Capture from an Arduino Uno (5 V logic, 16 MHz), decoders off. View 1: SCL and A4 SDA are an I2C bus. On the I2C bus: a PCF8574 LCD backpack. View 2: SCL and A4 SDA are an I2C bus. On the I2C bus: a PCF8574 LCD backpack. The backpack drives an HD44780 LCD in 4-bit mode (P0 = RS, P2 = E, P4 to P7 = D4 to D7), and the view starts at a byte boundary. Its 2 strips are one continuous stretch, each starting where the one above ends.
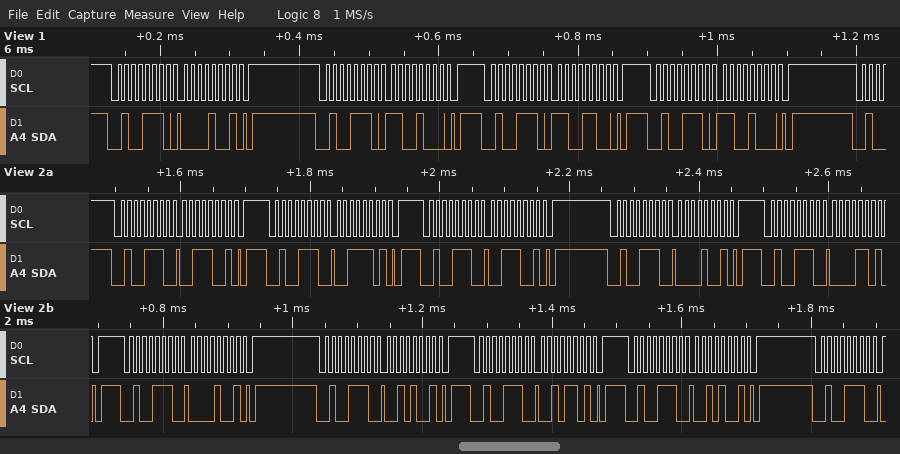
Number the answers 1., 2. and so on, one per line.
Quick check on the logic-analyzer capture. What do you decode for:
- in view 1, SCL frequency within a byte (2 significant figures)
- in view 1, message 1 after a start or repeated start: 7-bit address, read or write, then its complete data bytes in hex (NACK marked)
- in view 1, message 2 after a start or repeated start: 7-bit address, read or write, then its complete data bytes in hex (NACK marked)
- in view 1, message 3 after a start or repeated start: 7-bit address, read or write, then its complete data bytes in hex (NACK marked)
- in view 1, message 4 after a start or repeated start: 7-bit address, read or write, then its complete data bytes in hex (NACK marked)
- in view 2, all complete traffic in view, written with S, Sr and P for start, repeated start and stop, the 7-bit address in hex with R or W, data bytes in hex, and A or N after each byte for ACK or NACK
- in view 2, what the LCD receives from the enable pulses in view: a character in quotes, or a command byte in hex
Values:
1. 100 kHz
2. 0x27 write: 09
3. 0x27 write: C8
4. 0x27 write: CC
5. 0x27 write: C8
6. S 27W A 39 A P S 27W A 3D A P S 27W A 39 A P S 27W A 09 A P S 27W A 0D A P S 27W A 09 A P S 27W A 29 A P S 27W A 2D A P S 27W A 29 A P S 27W A
7. '0'
